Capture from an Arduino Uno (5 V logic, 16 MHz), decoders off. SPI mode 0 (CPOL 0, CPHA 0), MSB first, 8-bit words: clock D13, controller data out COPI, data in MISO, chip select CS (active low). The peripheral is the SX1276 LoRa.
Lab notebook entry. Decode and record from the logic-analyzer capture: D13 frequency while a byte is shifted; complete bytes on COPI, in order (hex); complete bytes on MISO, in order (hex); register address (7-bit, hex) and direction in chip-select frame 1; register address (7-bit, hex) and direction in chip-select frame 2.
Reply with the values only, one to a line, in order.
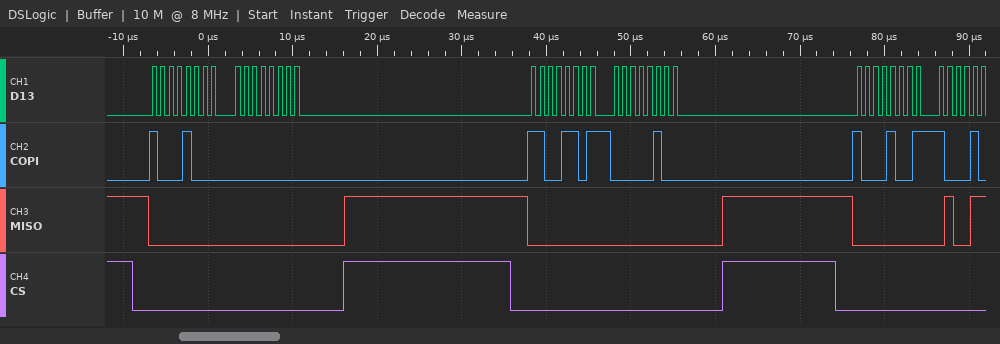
1 MHz
88 00 CD 04 89
00 00 00 00 00
0x08 write
0x4D write
